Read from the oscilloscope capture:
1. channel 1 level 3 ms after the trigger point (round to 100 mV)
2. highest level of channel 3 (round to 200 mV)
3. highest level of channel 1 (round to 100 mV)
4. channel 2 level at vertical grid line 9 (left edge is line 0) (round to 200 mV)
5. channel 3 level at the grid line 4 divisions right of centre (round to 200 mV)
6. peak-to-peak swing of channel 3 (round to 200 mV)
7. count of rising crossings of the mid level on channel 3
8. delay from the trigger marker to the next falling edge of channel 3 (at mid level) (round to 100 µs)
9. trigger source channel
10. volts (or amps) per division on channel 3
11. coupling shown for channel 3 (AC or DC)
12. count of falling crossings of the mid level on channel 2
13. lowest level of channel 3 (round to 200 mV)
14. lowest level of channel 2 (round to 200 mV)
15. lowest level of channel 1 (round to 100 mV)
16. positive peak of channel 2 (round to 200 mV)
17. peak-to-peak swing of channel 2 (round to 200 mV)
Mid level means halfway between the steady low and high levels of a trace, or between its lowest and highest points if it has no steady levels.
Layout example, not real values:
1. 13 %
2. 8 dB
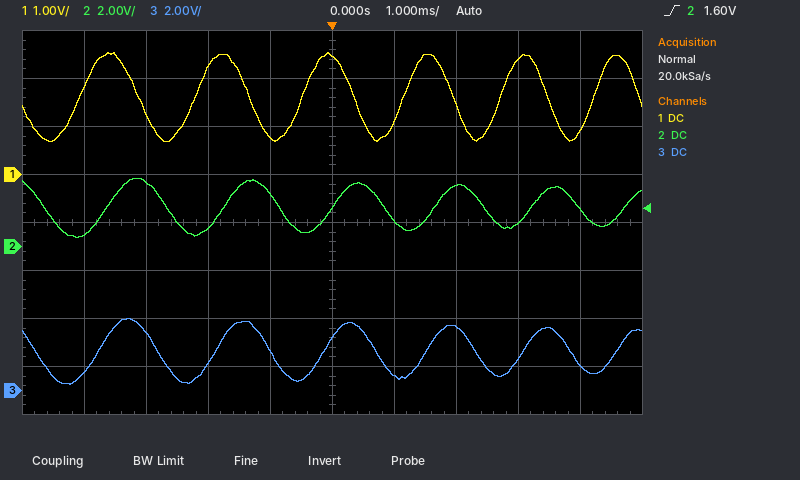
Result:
1. 2.4 V
2. 3.0 V
3. 2.5 V
4. 1.6 V
5. 1.0 V
6. 2.8 V
7. 6
8. 700 µs
9. channel 2
10. 2 V
11. DC
12. 6
13. 200 mV
14. 400 mV
15. 700 mV
16. 2.8 V
17. 2.4 V
